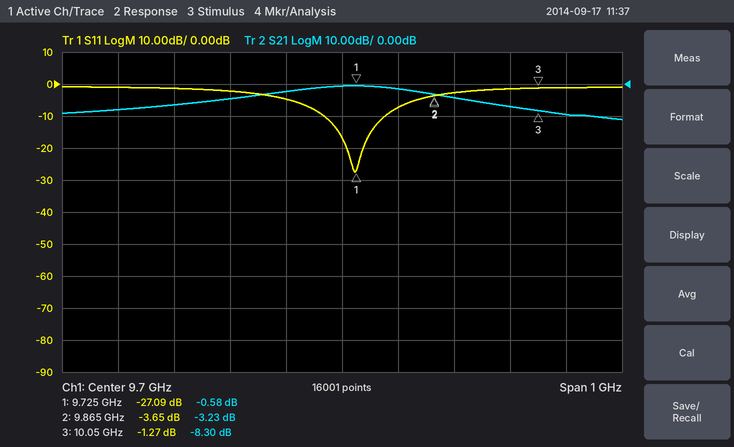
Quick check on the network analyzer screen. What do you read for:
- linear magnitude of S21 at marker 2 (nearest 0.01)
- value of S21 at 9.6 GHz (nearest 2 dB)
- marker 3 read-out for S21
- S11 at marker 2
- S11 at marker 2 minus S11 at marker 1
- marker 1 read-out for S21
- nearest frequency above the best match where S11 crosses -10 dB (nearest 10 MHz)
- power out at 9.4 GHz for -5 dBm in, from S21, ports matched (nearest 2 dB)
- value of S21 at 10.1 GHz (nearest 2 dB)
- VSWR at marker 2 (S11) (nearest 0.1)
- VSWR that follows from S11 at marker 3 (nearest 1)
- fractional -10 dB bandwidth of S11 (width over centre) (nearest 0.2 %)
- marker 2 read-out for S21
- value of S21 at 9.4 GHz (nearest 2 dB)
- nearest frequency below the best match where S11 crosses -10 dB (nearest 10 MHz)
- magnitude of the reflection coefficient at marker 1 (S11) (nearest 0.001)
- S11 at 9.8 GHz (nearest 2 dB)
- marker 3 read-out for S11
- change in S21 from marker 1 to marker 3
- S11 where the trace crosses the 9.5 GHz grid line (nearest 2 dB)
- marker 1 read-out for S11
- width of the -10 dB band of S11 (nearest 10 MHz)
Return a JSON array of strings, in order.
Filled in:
["0.69", "-2 dB", "-8.30 dB", "-3.65 dB", "23.44 dB", "-0.58 dB", "9.78 GHz", "-12 dBm", "-10 dB", "4.8", "14", "1.2 %", "-3.23 dB", "-6 dB", "9.67 GHz", "0.044", "-8 dB", "-1.27 dB", "-7.72 dB", "-2 dB", "-27.09 dB", "110 MHz"]
